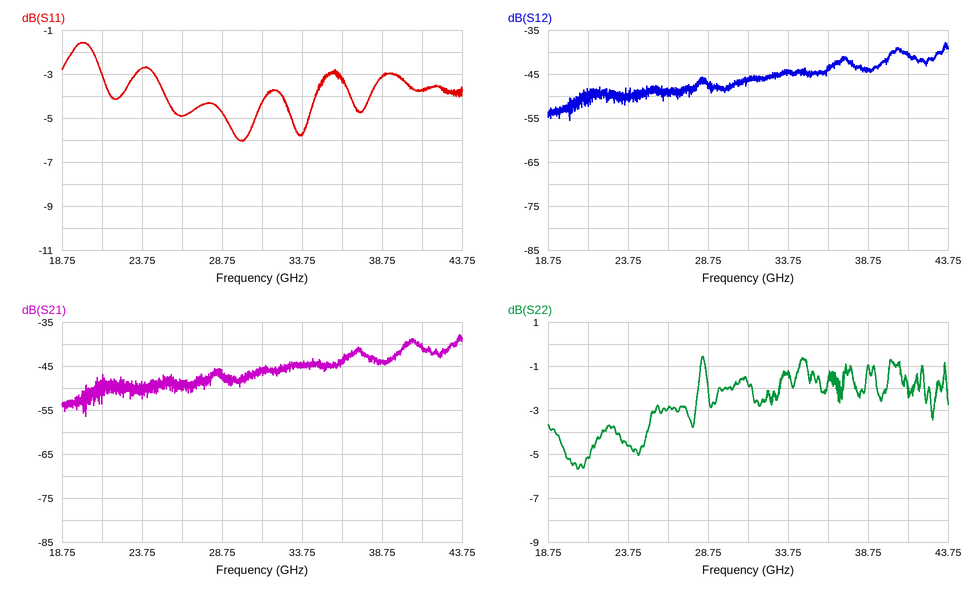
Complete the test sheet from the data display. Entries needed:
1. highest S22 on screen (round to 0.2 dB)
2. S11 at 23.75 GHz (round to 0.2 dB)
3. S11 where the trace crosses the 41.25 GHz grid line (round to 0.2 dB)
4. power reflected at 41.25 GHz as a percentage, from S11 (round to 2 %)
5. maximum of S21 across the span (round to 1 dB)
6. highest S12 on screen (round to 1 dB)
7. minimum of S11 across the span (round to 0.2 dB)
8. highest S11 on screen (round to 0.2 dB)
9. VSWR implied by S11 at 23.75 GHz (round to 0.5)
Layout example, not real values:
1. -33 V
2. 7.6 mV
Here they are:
1. -0.6 dB
2. -2.8 dB
3. -3.8 dB
4. 42 %
5. -38 dB
6. -38 dB
7. -6.0 dB
8. -1.6 dB
9. 6.5
